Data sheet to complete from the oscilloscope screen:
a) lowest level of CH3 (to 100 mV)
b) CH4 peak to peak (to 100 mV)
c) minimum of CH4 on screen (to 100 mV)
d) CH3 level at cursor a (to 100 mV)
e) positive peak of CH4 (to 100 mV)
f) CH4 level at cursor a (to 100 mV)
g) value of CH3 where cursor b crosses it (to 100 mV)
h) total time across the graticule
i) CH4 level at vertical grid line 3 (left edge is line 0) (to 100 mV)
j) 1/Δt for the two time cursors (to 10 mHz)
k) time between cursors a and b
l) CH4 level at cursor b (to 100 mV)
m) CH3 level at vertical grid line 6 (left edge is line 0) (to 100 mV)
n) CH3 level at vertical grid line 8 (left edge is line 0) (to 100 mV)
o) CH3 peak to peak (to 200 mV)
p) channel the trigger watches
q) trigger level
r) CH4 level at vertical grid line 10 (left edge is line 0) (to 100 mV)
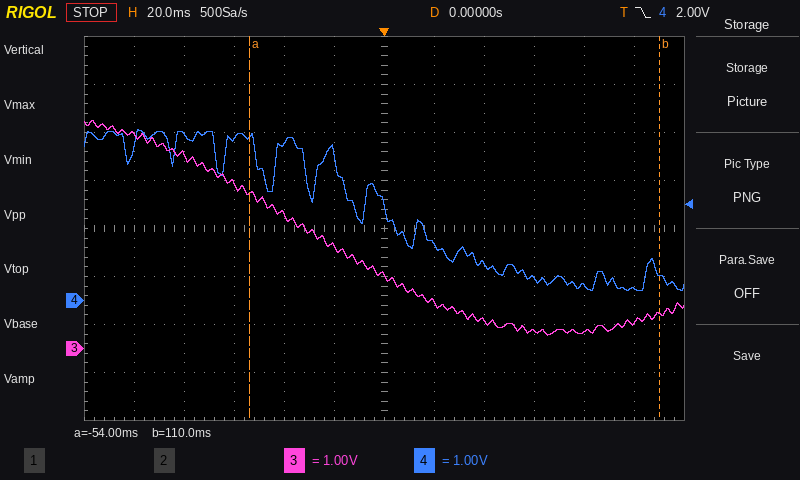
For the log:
300 mV
3.4 V
200 mV
3.2 V
3.6 V
3.4 V
700 mV
240 ms
3.4 V
6.10 Hz
164 ms
600 mV
1.5 V
600 mV
4.4 V
CH4
2.00 V
300 mV
